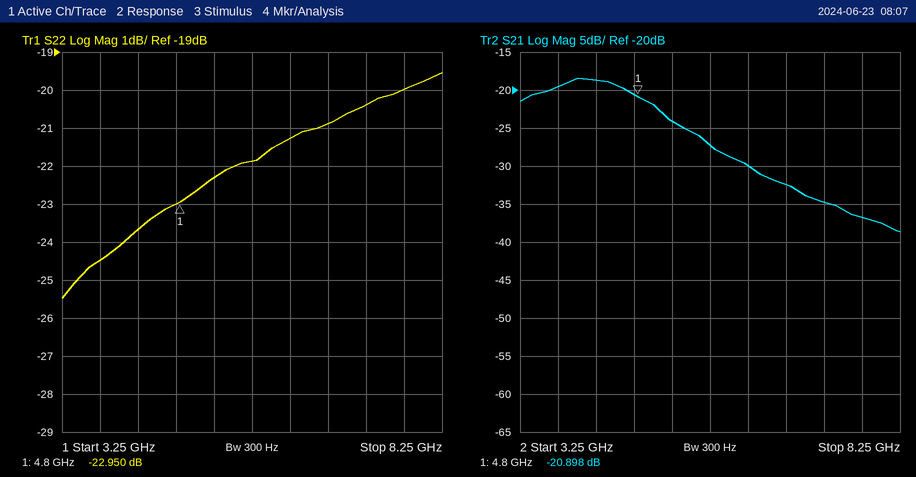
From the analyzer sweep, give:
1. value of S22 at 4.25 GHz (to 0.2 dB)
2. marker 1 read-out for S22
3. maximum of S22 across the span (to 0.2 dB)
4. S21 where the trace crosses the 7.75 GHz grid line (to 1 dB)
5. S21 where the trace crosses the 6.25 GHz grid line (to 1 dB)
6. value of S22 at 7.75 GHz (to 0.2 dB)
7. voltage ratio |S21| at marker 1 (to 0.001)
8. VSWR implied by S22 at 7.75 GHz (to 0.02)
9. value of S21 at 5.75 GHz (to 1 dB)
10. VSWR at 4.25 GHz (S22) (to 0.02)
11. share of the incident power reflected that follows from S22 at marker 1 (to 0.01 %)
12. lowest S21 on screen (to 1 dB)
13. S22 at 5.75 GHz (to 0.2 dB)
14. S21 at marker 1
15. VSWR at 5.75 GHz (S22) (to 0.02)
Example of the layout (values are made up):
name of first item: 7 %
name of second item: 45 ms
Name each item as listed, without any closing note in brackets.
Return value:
value of S22 at 4.25 GHz: -23.6 dB
marker 1 read-out for S22: -22.950 dB
maximum of S22 across the span: -19.6 dB
S21 where the trace crosses the 7.75 GHz grid line: -37 dB
S21 where the trace crosses the 6.25 GHz grid line: -30 dB
value of S22 at 7.75 GHz: -20.0 dB
voltage ratio |S21| at marker 1: 0.090
VSWR implied by S22 at 7.75 GHz: 1.22
value of S21 at 5.75 GHz: -27 dB
VSWR at 4.25 GHz (S22): 1.14
share of the incident power reflected that follows from S22 at marker 1: 0.51 %
lowest S21 on screen: -39 dB
S22 at 5.75 GHz: -21.8 dB
S21 at marker 1: -20.898 dB
VSWR at 5.75 GHz (S22): 1.18
